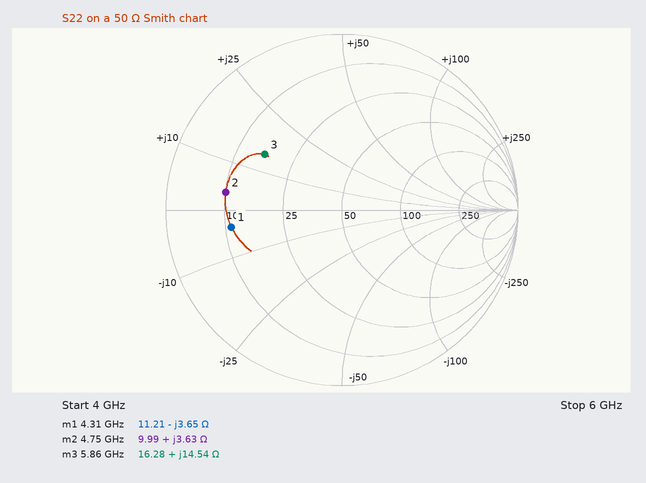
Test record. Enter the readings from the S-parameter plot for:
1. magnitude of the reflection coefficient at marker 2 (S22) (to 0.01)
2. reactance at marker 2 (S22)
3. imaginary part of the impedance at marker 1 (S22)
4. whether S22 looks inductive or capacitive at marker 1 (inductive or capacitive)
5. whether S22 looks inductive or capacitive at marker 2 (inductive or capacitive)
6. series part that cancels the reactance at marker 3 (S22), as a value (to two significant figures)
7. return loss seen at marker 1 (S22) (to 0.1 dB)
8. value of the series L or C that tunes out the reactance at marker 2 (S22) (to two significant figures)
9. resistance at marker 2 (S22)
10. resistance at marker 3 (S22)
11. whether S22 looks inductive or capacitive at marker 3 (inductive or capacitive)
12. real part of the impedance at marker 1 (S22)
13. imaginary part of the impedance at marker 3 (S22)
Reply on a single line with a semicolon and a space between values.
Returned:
0.67; +3.63 Ω; -3.65 Ω; capacitive; inductive; 1.9 pF; 3.9 dB; 9.2 pF; 9.99 Ω; 16.28 Ω; inductive; 11.21 Ω; +14.54 Ω
